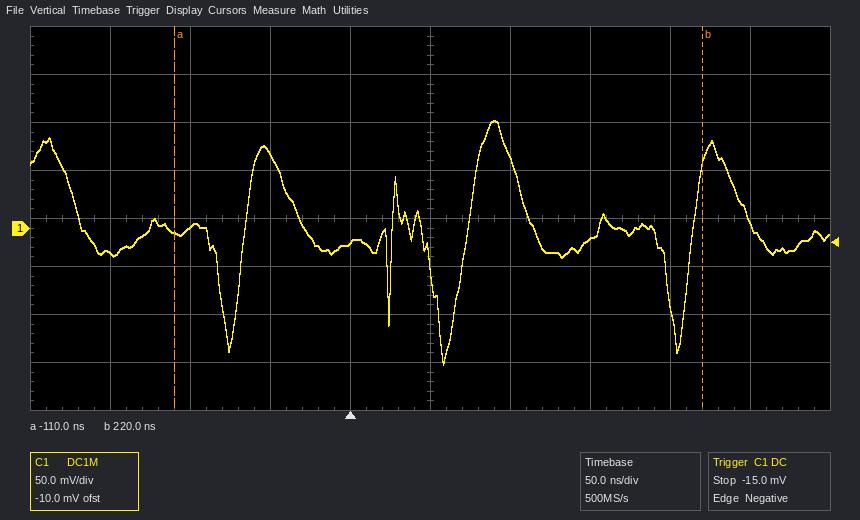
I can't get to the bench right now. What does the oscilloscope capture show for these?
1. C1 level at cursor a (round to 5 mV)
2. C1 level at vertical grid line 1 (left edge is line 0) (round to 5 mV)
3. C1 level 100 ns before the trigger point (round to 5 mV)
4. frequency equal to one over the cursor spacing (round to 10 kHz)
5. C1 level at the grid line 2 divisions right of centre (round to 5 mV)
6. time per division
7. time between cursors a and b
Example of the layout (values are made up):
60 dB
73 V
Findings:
-5 mV
-25 mV
0 mV
3.03 MHz
-10 mV
50 ns
330 ns
